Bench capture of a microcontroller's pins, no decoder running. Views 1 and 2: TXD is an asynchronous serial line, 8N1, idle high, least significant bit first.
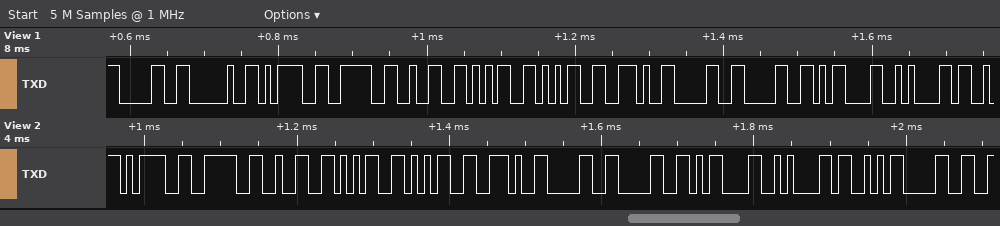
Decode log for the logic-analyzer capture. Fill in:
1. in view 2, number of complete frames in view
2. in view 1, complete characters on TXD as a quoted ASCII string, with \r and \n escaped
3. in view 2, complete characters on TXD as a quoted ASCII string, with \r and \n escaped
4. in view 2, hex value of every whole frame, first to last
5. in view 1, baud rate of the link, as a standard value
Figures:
12
"0 =>255.00\r\n"
"=>255.00\r\nS0"
3D 3E 32 35 35 2E 30 30 0D 0A 53 30
115200 baud
